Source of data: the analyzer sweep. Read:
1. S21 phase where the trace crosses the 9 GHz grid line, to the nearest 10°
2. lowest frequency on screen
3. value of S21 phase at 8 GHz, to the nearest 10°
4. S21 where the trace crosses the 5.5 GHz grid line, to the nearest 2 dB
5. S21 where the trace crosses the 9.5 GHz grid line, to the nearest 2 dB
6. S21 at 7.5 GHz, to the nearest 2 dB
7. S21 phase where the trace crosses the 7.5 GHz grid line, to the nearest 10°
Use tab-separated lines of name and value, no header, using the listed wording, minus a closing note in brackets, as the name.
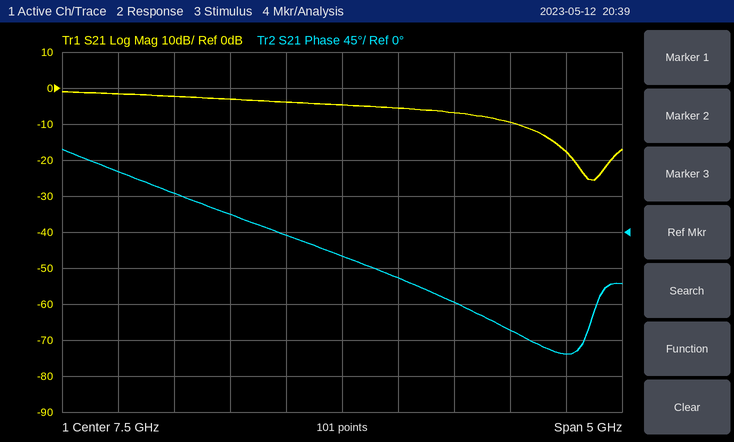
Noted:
S21 phase where the trace crosses the 9 GHz grid line, to the nearest 10°	-120°
lowest frequency on screen	5 GHz
value of S21 phase at 8 GHz, to the nearest 10°	-60°
S21 where the trace crosses the 5.5 GHz grid line, to the nearest 2 dB	-2 dB
S21 where the trace crosses the 9.5 GHz grid line, to the nearest 2 dB	-18 dB
S21 at 7.5 GHz, to the nearest 2 dB	-4 dB
S21 phase where the trace crosses the 7.5 GHz grid line, to the nearest 10°	-30°
